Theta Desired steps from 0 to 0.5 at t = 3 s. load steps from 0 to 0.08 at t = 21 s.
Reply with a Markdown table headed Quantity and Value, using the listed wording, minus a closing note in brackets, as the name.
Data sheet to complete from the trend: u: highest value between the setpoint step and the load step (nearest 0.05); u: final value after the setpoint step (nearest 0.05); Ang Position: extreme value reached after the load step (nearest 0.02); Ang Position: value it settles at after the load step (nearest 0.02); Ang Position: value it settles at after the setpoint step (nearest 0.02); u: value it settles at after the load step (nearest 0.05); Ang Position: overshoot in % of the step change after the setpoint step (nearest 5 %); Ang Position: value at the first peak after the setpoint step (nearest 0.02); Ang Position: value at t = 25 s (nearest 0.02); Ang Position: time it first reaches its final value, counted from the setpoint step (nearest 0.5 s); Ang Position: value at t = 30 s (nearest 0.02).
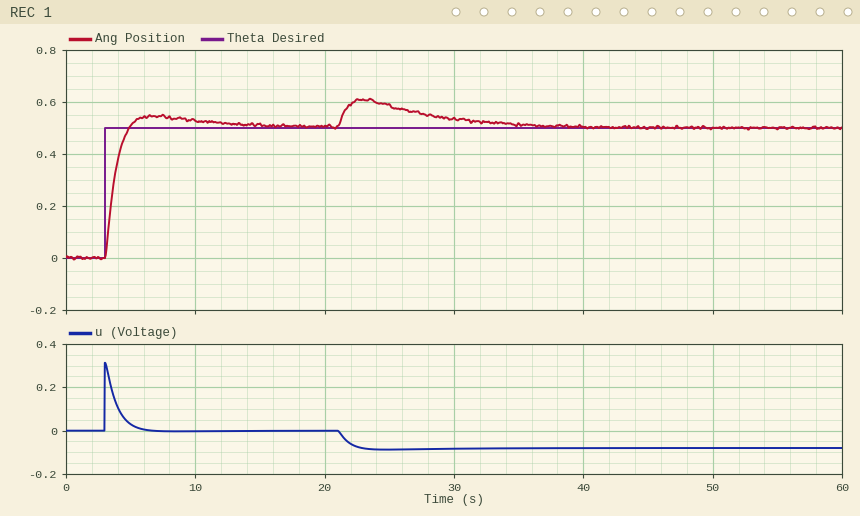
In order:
| Quantity | Value |
|---|---|
| u: highest value between the setpoint step and the load step | 0.30 |
| u: final value after the setpoint step | 0.00 |
| Ang Position: extreme value reached after the load step | 0.60 |
| Ang Position: value it settles at after the load step | 0.50 |
| Ang Position: value it settles at after the setpoint step | 0.50 |
| u: value it settles at after the load step | -0.10 |
| Ang Position: overshoot in % of the step change after the setpoint step | 10 % |
| Ang Position: value at the first peak after the setpoint step | 0.54 |
| Ang Position: value at t = 25 s | 0.58 |
| Ang Position: time it first reaches its final value, counted from the setpoint step | 2.0 s |
| Ang Position: value at t = 30 s | 0.54 |
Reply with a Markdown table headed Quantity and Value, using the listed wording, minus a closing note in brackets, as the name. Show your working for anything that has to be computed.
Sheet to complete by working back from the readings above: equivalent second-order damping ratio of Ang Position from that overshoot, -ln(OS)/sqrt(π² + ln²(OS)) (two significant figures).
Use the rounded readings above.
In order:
| Quantity | Value |
|---|---|
| equivalent second-order damping ratio of Ang Position from that overshoot, -ln(OS)/sqrt(π² + ln²(OS)) | ln(0.1) = -2.303; 2.303 / sqrt(9.870 + 5.302) = 0.59 |
